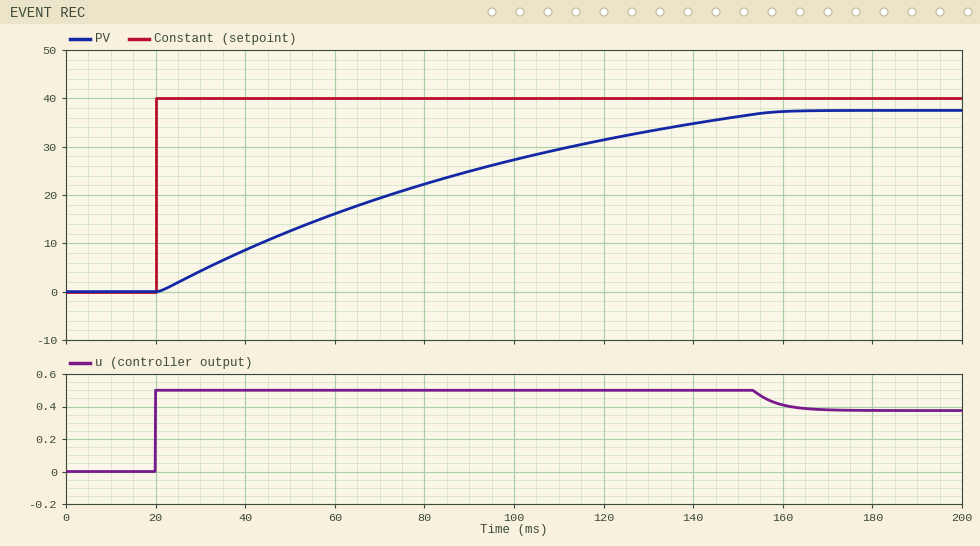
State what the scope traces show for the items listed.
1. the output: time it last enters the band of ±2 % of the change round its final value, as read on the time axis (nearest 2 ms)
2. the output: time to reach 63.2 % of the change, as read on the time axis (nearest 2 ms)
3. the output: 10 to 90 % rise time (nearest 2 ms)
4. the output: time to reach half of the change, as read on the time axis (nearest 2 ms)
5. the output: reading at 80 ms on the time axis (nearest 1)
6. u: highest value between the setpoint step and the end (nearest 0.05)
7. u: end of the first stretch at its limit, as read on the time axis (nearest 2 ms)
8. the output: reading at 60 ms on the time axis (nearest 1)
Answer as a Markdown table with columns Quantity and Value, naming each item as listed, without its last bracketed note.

| Quantity | Value |
|---|---|
| the output: time it last enters the band of ±2 % of the change round its final value, as read on the time axis | 154 ms |
| the output: time to reach 63.2 % of the change, as read on the time axis | 86 ms |
| the output: 10 to 90 % rise time | 104 ms |
| the output: time to reach half of the change, as read on the time axis | 68 ms |
| the output: reading at 80 ms on the time axis | 22 |
| u: highest value between the setpoint step and the end | 0.50 |
| u: end of the first stretch at its limit, as read on the time axis | 154 ms |
| the output: reading at 60 ms on the time axis | 16 |
